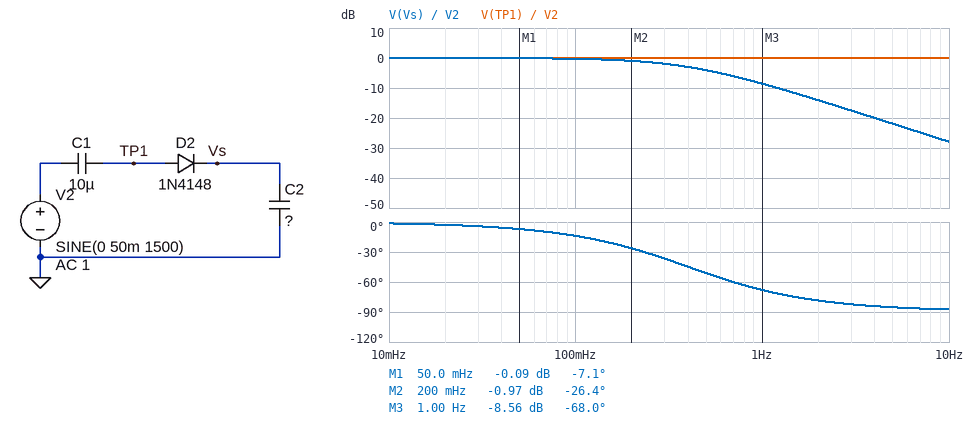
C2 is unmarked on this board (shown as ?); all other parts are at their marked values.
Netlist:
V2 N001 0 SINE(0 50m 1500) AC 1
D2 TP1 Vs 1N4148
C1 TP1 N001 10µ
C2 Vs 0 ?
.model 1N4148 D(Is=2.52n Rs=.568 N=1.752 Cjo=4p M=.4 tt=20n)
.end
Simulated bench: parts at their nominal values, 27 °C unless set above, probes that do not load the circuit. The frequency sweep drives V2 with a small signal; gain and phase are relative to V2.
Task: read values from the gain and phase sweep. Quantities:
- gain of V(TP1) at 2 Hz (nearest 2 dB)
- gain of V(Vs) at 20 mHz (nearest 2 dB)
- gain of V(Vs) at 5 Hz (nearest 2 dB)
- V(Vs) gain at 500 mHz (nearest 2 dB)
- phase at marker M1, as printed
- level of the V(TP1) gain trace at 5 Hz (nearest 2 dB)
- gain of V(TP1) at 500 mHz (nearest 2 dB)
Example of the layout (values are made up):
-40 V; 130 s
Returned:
0 dB; 0 dB; -22 dB; -4 dB; -7.1 deg; 0 dB; 0 dB
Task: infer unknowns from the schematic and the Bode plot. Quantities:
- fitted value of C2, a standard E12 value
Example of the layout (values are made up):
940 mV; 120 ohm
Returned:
22 nF
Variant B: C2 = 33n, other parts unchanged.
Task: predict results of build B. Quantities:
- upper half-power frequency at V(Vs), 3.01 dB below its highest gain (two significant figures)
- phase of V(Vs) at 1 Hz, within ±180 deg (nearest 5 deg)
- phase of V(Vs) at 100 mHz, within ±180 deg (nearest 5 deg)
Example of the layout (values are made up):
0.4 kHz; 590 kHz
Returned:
270 mHz; -75 deg; -20 deg
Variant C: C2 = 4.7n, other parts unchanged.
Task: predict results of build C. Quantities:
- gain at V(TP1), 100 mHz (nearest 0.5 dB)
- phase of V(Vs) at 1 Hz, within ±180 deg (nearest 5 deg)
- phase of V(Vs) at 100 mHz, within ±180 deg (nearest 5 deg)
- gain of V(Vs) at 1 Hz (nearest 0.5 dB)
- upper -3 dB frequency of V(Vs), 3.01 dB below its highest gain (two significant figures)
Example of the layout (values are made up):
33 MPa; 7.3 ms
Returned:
0 dB; -30 deg; -5 deg; -1.0 dB; 1.9 Hz
